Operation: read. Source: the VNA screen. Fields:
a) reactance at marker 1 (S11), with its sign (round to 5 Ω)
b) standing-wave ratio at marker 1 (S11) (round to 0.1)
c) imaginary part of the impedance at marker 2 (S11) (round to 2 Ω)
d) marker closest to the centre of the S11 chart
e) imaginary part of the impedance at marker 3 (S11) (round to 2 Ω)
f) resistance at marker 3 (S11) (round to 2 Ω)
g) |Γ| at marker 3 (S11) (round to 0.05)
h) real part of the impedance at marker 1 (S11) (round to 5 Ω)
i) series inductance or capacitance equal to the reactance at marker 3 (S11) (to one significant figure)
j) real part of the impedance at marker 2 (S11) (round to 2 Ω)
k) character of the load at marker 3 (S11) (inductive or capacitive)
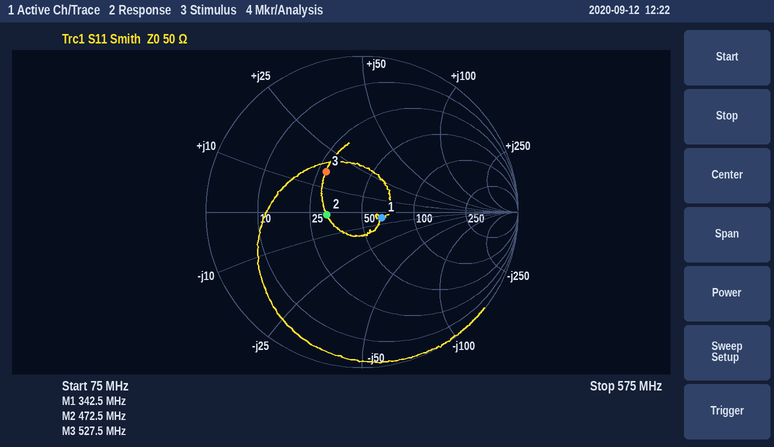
-5 Ω
1.3
-2 Ω
marker 1
+16 Ω
28 Ω
0.35
65 Ω
5 nH
32 Ω
inductive
